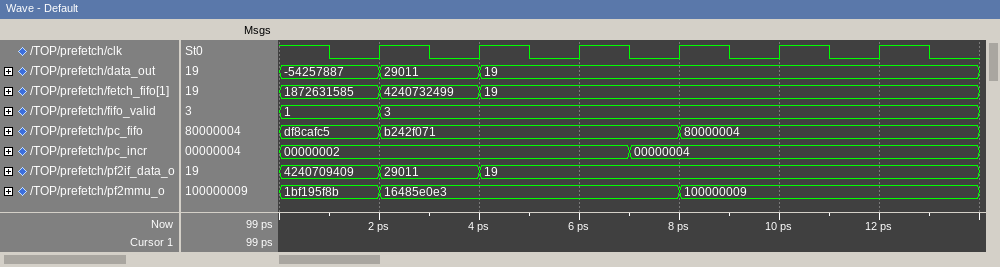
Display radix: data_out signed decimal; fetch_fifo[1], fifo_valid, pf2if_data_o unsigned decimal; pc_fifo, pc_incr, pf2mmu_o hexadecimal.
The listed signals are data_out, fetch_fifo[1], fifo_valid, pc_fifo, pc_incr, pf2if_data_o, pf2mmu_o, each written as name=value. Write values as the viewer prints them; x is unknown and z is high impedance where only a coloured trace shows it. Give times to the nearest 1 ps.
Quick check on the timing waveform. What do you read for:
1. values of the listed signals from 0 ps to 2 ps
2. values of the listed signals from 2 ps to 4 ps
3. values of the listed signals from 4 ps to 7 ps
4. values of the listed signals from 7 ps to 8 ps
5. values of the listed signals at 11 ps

data_out=-54257887, fetch_fifo[1]=1872631585, fifo_valid=1, pc_fifo=df8cafc5, pc_incr=00000002, pf2if_data_o=4240709409, pf2mmu_o=1bf195f8b
data_out=29011, fetch_fifo[1]=4240732499, fifo_valid=3, pc_fifo=b242f071, pc_incr=00000002, pf2if_data_o=29011, pf2mmu_o=16485e0e3
data_out=19, fetch_fifo[1]=19, fifo_valid=3, pc_fifo=b242f071, pc_incr=00000002, pf2if_data_o=19, pf2mmu_o=16485e0e3
data_out=19, fetch_fifo[1]=19, fifo_valid=3, pc_fifo=b242f071, pc_incr=00000004, pf2if_data_o=19, pf2mmu_o=16485e0e3
data_out=19, fetch_fifo[1]=19, fifo_valid=3, pc_fifo=80000004, pc_incr=00000004, pf2if_data_o=19, pf2mmu_o=100000009
